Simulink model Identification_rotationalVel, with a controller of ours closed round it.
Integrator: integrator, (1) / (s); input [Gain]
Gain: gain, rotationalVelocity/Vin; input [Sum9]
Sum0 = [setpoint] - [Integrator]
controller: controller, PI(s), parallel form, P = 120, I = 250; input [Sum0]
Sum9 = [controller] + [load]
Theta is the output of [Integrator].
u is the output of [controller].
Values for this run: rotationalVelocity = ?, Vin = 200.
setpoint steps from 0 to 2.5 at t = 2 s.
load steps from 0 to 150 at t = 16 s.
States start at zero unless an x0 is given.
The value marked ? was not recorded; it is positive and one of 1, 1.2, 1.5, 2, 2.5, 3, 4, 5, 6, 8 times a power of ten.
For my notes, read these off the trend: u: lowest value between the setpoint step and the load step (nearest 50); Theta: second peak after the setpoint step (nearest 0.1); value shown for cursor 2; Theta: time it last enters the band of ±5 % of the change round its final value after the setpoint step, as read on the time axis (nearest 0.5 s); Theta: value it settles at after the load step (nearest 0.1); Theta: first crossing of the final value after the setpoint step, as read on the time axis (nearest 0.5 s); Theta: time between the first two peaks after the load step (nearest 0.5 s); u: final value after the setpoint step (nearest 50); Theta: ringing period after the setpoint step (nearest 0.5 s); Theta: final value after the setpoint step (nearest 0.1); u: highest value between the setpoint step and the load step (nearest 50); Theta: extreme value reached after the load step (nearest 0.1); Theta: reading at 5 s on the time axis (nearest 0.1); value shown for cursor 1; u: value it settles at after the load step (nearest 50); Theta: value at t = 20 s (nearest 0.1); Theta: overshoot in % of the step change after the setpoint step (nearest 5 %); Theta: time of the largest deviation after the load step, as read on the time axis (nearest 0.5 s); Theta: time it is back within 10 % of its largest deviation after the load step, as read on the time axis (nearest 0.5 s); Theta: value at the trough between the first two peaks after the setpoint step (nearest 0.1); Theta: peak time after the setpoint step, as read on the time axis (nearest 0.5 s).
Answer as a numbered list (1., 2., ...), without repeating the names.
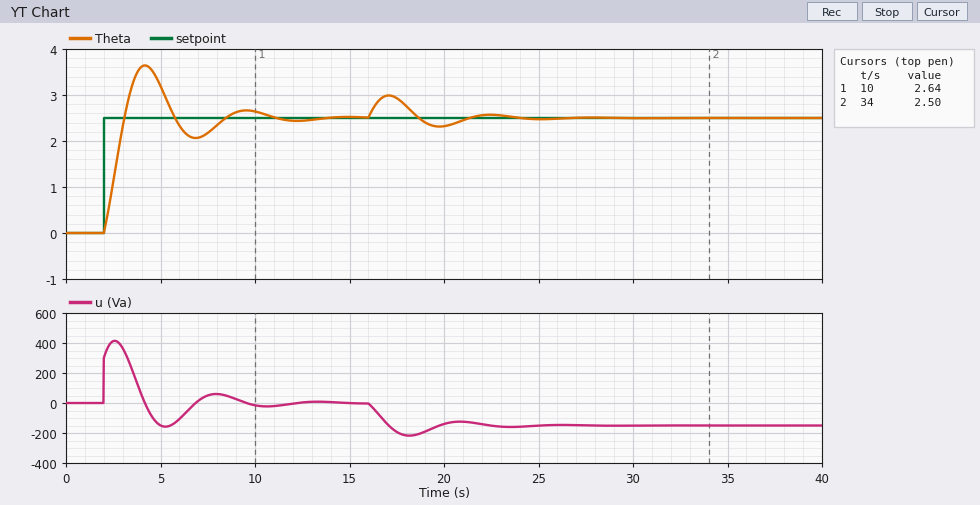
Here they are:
1. -150
2. 2.7
3. 2.50
4. 10.0 s
5. 2.5
6. 3.0 s
7. 5.5 s
8. 0
9. 5.5 s
10. 2.5
11. 400
12. 3.0
13. 3.2
14. 2.64
15. -150
16. 2.3
17. 45 %
18. 17.0 s
19. 23.0 s
20. 2.1
21. 4.0 s
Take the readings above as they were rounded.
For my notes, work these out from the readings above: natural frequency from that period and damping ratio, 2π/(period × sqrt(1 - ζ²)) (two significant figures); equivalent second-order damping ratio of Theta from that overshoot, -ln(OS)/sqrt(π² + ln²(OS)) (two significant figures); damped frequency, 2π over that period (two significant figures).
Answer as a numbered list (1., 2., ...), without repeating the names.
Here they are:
1. 1.2 rad/s
2. 0.25
3. 1.1 rad/s
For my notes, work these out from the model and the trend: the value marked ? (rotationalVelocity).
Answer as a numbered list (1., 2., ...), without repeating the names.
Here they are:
1. 1.2
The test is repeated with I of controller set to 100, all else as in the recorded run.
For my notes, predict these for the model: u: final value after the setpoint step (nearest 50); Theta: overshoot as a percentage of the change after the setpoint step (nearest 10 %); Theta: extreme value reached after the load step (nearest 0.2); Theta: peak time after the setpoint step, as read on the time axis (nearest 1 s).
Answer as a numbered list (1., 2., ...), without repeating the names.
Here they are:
1. 0
2. 30 %
3. 3.2
4. 5 s
